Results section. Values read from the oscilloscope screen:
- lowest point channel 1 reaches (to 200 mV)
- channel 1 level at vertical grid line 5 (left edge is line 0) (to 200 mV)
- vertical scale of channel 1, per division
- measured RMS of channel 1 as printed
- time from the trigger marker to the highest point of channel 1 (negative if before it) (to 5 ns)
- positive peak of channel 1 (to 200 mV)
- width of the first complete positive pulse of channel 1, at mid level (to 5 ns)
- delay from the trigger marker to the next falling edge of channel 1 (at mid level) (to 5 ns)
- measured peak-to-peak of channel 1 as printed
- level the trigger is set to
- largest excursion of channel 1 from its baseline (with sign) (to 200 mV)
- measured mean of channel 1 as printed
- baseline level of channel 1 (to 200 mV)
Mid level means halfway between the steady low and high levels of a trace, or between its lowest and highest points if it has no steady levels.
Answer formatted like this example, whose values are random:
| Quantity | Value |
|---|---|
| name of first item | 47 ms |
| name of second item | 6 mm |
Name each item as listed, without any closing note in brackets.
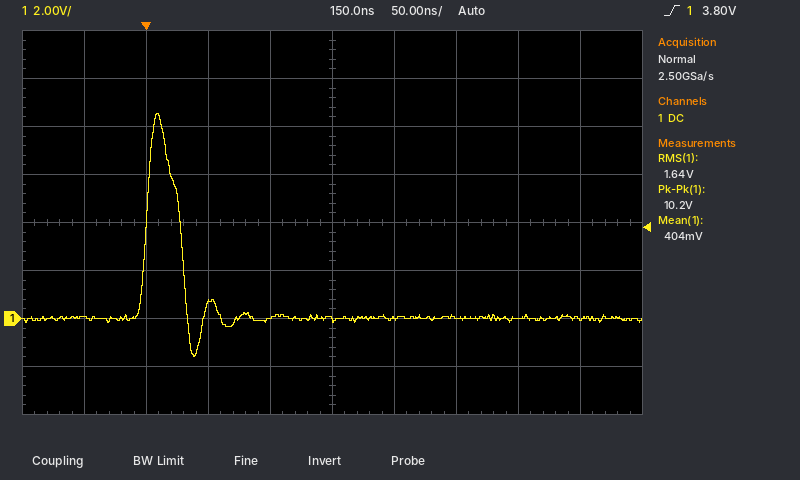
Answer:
| Quantity | Value |
|---|---|
| lowest point channel 1 reaches | -1.6 V |
| channel 1 level at vertical grid line 5 (left edge is line 0) | 0.0 V |
| vertical scale of channel 1, per division | 2 V |
| measured RMS of channel 1 as printed | 1.64 V |
| time from the trigger marker to the highest point of channel 1 (negative if before it) | +10 ns |
| positive peak of channel 1 | 8.6 V |
| width of the first complete positive pulse of channel 1, at mid level | 30 ns |
| delay from the trigger marker to the next falling edge of channel 1 (at mid level) | 30 ns |
| measured peak-to-peak of channel 1 as printed | 10.2 V |
| level the trigger is set to | 3.80 V |
| largest excursion of channel 1 from its baseline (with sign) | +8.6 V |
| measured mean of channel 1 as printed | 404 mV |
| baseline level of channel 1 | 0.0 V |
